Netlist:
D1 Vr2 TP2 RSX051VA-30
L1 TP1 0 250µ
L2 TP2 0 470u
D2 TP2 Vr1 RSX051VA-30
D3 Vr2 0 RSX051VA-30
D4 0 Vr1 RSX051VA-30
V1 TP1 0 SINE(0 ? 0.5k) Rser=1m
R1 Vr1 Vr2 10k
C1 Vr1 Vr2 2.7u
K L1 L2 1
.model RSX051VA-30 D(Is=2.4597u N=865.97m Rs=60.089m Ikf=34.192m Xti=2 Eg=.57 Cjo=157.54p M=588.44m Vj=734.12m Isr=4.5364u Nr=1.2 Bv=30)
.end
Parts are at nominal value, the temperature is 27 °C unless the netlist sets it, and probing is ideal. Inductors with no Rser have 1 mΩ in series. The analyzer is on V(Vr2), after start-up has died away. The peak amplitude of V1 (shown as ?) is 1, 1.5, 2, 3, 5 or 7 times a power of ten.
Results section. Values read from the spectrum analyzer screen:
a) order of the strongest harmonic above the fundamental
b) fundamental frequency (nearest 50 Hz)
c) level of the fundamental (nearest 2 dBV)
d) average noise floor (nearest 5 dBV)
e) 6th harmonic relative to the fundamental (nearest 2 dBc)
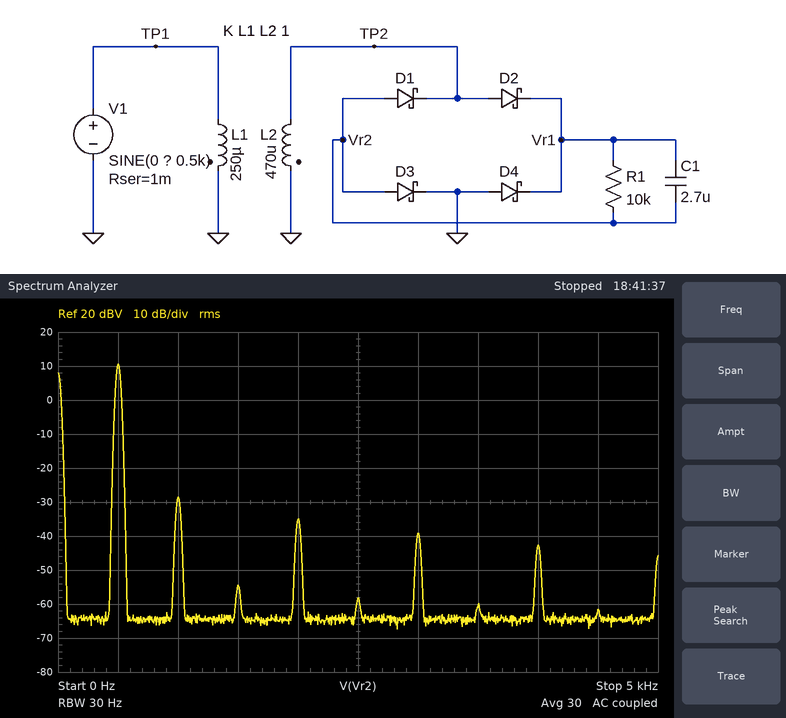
2
500 Hz
10 dBV
-65 dBV
-50 dBc
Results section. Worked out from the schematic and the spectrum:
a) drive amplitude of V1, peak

7 V
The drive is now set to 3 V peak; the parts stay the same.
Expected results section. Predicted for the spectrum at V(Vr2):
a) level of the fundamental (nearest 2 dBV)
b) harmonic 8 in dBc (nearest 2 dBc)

4 dBV
-56 dBc
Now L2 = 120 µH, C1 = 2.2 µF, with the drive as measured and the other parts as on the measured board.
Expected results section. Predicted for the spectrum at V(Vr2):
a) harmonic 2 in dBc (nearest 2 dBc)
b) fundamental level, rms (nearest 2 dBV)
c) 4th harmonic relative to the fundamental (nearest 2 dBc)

-38 dBc
4 dBV
-44 dBc
